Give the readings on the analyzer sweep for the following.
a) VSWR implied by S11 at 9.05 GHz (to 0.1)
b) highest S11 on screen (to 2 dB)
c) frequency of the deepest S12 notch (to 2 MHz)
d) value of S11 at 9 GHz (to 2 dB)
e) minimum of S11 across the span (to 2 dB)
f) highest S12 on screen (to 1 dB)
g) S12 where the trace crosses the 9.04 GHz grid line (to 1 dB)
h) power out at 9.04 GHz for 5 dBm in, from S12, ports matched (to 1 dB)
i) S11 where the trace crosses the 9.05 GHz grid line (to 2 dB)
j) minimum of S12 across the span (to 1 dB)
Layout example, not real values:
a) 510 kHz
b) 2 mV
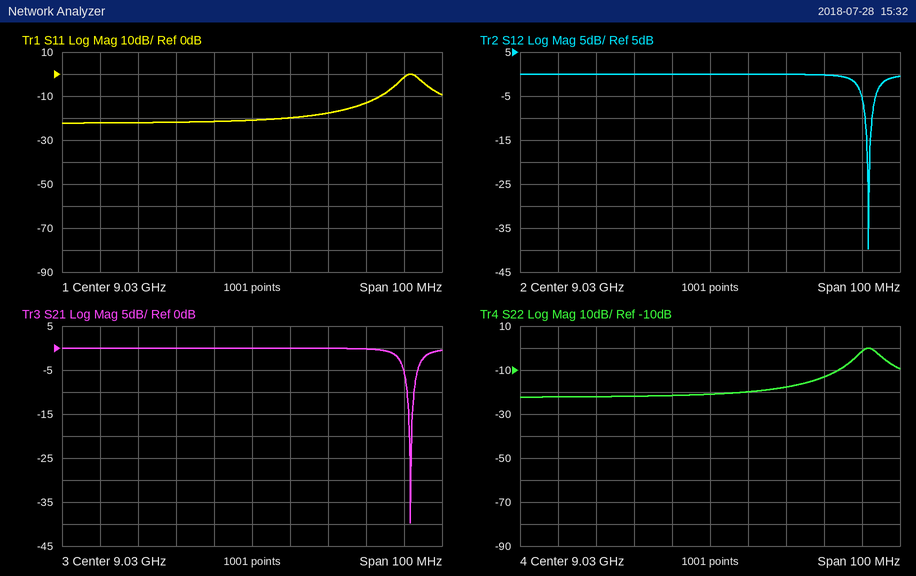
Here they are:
a) 1.3
b) 0 dB
c) 9.072 GHz
d) -22 dB
e) -22 dB
f) 0 dB
g) 0 dB
h) 5 dBm
i) -18 dB
j) -40 dB
